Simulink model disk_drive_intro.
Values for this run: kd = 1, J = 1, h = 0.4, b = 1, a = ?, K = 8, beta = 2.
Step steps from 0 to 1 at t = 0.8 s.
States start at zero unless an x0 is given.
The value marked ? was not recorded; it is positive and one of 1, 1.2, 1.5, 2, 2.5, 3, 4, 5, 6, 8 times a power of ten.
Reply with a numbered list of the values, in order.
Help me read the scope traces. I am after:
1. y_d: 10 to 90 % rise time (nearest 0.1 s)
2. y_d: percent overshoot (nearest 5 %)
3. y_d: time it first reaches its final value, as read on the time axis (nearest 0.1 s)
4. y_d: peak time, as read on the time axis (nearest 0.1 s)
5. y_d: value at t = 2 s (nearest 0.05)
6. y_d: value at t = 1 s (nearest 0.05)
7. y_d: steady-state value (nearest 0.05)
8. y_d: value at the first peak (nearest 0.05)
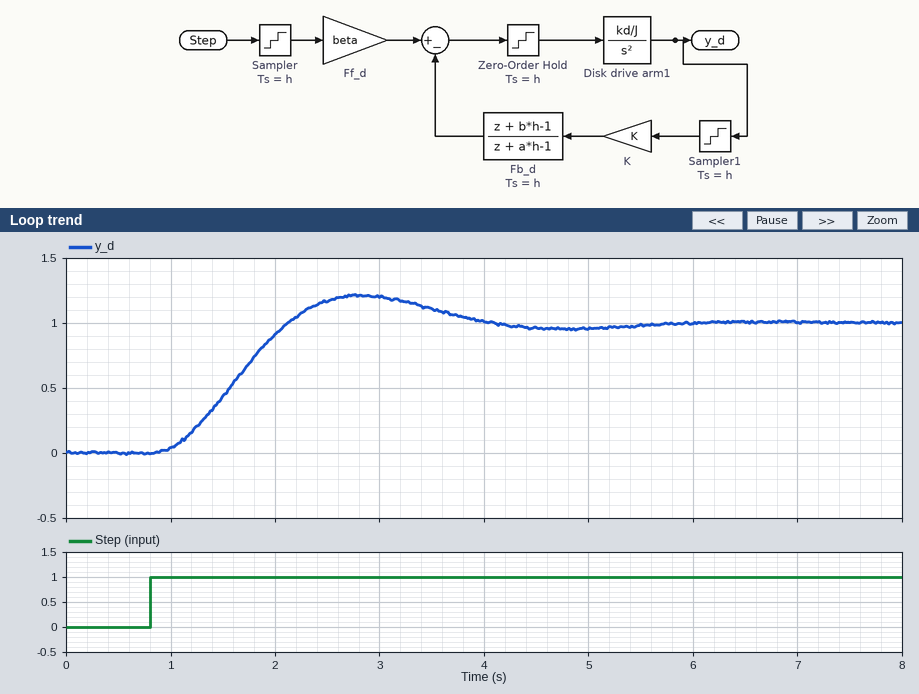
1. 0.9 s
2. 20 %
3. 2.1 s
4. 2.8 s
5. 0.90
6. 0.05
7. 1.00
8. 1.20
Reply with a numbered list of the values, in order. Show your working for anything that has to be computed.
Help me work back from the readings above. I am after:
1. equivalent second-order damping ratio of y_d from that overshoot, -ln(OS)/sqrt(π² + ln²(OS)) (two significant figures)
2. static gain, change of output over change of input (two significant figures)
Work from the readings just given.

1. ln(0.2) = -1.609; 1.609 / sqrt(9.870 + 2.590) = 0.46
2. (1 - 0) / (1 - 0) = 1.0
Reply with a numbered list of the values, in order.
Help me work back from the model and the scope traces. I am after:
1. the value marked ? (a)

1. 4
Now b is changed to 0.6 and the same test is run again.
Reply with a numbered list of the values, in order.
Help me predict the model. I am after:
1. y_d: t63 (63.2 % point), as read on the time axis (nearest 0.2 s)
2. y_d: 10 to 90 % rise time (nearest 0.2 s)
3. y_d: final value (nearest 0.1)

1. 2.2 s
2. 1.8 s
3. 1.7
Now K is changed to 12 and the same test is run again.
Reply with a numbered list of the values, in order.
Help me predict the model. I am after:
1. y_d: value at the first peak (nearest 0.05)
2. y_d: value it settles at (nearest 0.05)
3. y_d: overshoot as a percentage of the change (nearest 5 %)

1. 0.75
2. 0.65
3. 10 %
